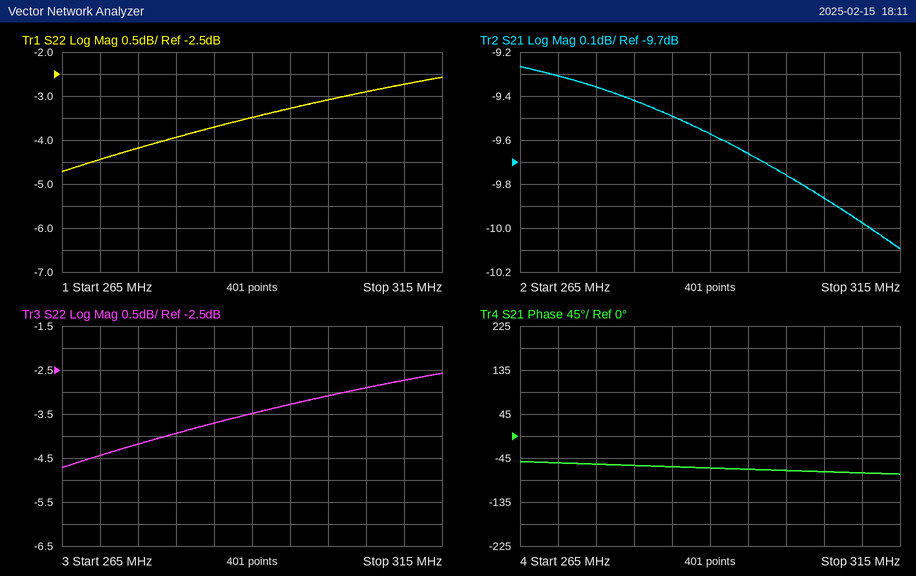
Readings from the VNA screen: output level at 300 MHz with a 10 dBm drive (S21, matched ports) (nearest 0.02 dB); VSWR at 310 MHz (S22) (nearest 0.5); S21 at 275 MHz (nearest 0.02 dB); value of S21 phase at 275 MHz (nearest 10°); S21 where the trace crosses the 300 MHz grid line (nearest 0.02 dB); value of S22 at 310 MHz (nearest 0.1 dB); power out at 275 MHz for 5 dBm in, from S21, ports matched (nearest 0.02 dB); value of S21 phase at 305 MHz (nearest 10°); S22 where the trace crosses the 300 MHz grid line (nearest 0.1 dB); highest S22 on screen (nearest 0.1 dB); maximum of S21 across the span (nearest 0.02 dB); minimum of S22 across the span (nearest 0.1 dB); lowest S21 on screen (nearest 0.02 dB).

0.24 dBm
6.5
-9.36 dB
-60°
-9.76 dB
-2.7 dB
-4.36 dBm
-70°
-3.1 dB
-2.6 dB
-9.26 dB
-4.7 dB
-10.10 dB
